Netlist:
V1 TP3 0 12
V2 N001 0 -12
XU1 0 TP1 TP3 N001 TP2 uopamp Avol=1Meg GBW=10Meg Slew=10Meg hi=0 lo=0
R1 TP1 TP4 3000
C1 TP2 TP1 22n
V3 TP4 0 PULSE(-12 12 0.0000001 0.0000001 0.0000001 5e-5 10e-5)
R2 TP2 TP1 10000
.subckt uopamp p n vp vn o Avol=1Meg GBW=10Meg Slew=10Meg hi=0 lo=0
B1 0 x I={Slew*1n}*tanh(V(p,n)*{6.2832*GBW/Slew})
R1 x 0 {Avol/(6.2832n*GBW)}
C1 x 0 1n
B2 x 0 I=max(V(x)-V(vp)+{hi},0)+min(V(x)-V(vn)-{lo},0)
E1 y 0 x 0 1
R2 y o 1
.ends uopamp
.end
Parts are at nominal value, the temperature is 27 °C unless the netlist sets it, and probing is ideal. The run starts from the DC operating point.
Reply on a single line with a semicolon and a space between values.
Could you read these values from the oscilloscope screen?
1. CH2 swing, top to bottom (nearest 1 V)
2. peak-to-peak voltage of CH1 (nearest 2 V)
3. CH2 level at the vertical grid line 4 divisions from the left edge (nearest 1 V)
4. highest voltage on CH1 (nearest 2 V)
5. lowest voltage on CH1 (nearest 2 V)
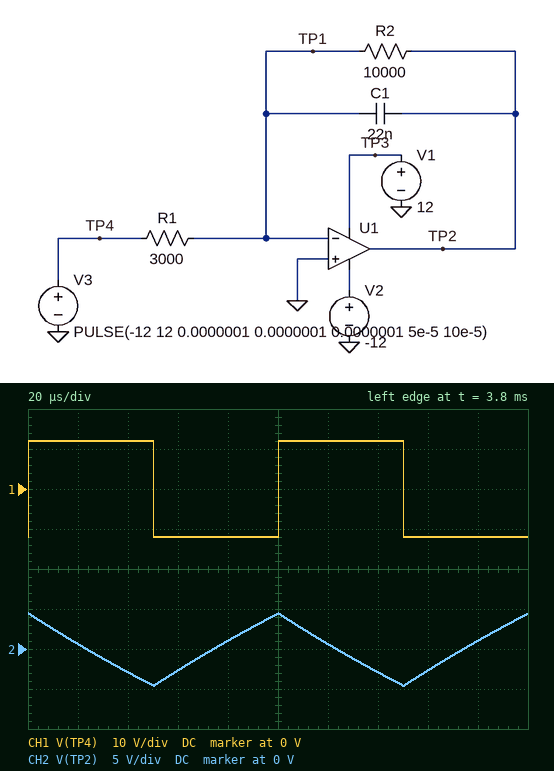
9 V; 24 V; 1 V; 12 V; -12 V
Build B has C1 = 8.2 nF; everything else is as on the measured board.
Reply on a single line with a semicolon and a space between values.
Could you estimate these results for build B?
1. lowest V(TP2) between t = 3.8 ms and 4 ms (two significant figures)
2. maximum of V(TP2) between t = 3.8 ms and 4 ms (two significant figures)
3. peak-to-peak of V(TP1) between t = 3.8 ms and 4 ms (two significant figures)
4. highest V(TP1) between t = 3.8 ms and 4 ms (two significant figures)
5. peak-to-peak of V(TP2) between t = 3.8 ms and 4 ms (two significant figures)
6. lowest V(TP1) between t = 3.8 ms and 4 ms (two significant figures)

-12 V; 12 V; 20 mV; 10 mV; 24 V; -10 mV
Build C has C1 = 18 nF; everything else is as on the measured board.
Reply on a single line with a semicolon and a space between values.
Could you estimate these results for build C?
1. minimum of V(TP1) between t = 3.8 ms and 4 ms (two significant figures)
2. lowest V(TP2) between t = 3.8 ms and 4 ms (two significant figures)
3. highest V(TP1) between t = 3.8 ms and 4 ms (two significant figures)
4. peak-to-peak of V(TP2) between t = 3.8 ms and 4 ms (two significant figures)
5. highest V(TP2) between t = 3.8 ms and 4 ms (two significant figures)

-4.2 mV; -5.6 V; 4.2 mV; 11 V; 5.4 V
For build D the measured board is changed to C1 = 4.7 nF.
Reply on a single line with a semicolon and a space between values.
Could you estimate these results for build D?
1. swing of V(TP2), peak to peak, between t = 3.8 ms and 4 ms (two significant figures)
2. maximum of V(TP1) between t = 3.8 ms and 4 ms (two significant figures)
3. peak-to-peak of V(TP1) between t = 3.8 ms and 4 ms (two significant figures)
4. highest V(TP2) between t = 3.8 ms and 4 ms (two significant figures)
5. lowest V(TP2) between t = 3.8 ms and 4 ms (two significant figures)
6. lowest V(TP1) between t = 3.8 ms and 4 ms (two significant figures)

24 V; 5.1 V; 10 V; 12 V; -12 V; -5.1 V
